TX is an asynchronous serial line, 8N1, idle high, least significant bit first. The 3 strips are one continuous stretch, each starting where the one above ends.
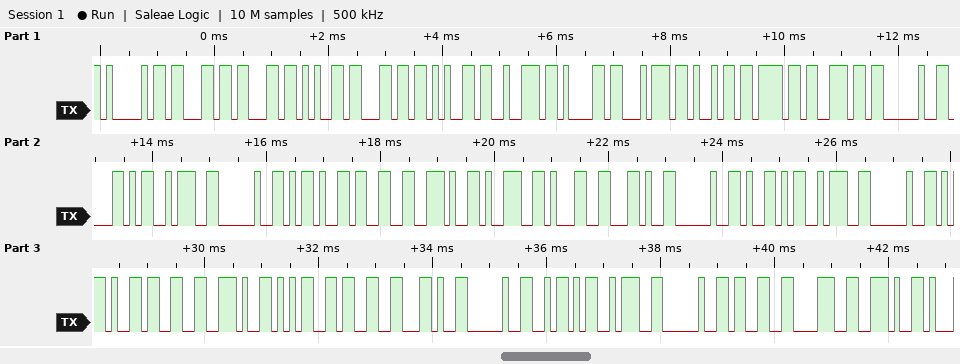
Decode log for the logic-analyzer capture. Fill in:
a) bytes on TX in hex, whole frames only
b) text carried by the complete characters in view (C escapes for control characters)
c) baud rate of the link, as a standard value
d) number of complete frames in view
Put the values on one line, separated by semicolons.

41 63 63 65 6C 65 72 61 74 69 6F 6E 20 58 3A 20 2D 33 2E 39 31 2C 20 59 3A 20 2D 33 2E 35 33 2C 20 5A 3A 20 33 38 2E; "Acceleration X: -3.91, Y: -3.53, Z: 38."; 9600 baud; 39
